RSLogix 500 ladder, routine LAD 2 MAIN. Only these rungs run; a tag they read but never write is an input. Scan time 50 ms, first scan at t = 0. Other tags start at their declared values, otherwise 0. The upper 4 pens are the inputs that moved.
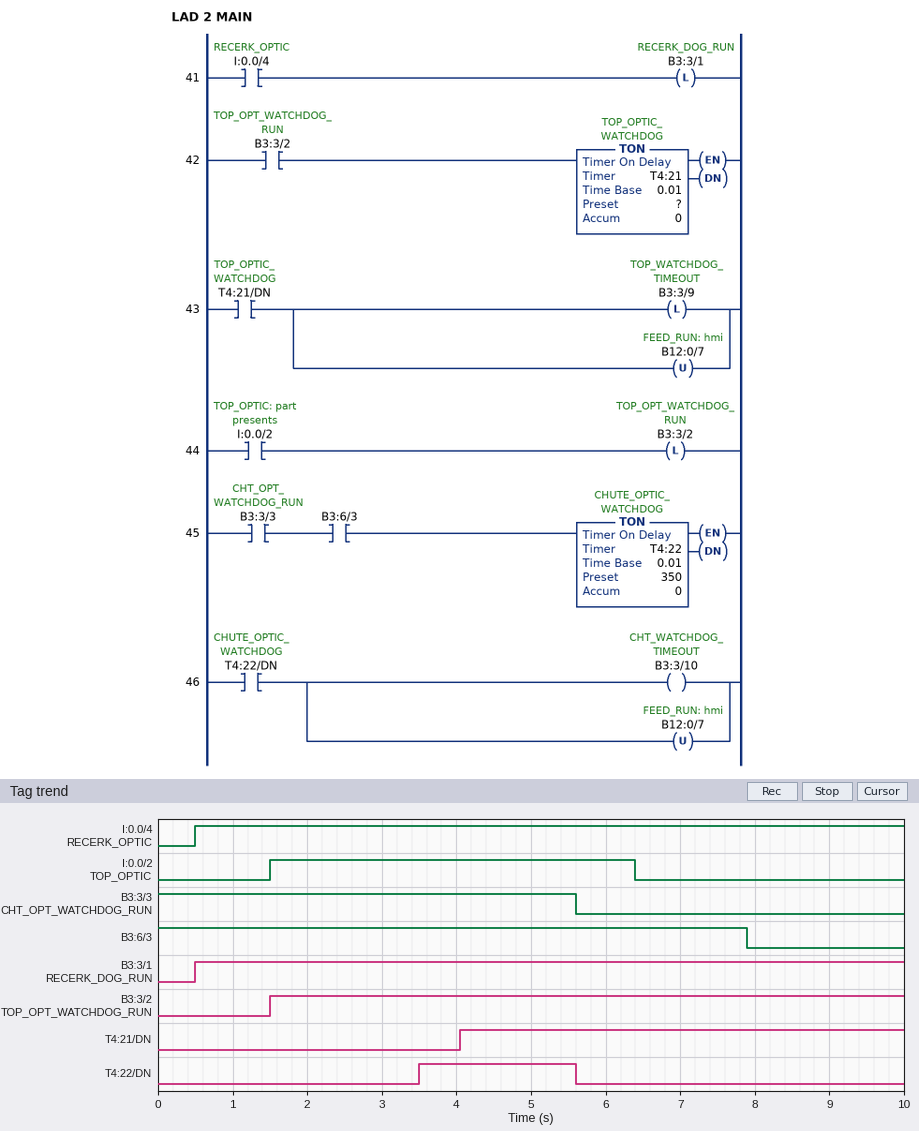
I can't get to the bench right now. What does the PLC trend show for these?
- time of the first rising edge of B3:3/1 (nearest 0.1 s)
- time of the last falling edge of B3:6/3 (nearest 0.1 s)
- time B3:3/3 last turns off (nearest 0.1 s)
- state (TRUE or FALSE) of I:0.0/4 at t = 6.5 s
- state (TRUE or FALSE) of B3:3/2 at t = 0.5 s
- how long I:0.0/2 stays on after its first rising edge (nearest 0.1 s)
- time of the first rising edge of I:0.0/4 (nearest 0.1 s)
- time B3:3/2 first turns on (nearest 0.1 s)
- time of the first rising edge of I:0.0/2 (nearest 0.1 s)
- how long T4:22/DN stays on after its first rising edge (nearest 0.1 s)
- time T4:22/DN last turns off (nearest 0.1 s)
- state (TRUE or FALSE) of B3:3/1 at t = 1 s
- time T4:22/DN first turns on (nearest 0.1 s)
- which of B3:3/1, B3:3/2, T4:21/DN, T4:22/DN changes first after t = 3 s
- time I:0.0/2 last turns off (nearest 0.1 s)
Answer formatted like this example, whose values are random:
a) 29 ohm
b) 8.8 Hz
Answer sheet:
a) 0.5 s
b) 7.9 s
c) 5.6 s
d) TRUE
e) FALSE
f) 4.9 s
g) 0.5 s
h) 1.5 s
i) 1.5 s
j) 2.1 s
k) 5.6 s
l) TRUE
m) 3.5 s
n) T4:22/DN
o) 6.4 s
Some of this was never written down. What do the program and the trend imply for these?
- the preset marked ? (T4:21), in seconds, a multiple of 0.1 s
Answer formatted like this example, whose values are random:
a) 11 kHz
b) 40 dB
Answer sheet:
a) 2.5 s
